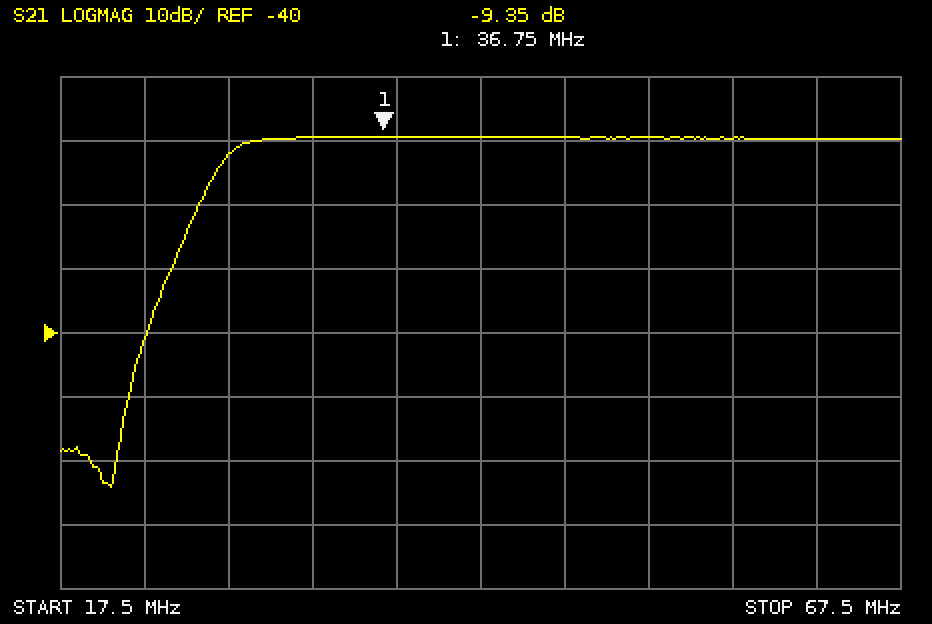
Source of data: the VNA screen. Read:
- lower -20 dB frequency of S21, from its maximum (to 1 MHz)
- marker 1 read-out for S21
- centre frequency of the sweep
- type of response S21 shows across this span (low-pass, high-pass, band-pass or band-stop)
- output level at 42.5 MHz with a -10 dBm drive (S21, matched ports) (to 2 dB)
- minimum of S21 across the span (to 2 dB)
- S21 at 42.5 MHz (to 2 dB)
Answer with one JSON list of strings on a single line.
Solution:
["24 MHz", "-9.35 dB", "42.5 MHz", "high-pass", "-20 dBm", "-64 dB", "-10 dB"]
